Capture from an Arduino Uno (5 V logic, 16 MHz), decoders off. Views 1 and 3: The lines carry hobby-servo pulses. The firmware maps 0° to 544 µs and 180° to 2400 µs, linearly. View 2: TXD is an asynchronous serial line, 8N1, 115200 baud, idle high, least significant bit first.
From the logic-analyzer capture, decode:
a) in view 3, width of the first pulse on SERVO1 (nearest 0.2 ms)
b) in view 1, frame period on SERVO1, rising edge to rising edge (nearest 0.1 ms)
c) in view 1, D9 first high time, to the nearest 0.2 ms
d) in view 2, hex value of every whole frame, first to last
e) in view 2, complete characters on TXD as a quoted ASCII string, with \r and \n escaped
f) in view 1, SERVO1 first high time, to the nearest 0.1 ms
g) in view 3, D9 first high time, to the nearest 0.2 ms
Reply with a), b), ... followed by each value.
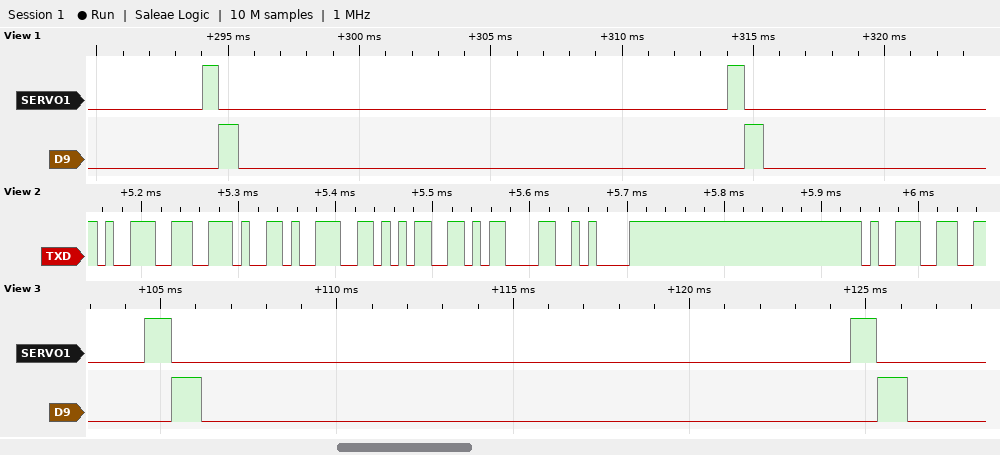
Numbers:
a) 0.8 ms
b) 20.0 ms
c) 0.8 ms
d) 39 2E 39 35 0D 0A 39
e) "9.95\r\n9"
f) 0.6 ms
g) 0.8 ms
